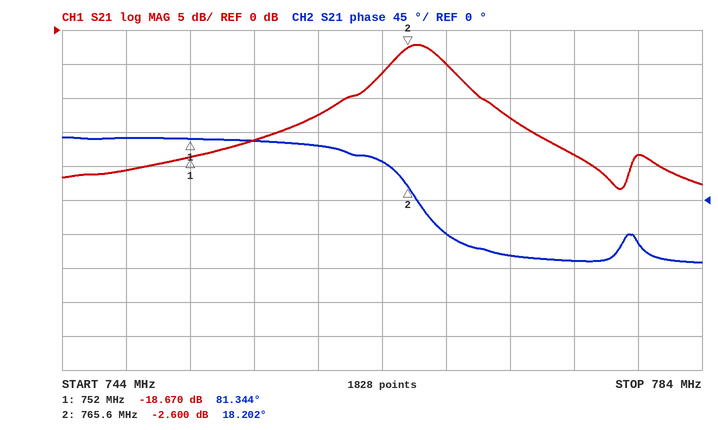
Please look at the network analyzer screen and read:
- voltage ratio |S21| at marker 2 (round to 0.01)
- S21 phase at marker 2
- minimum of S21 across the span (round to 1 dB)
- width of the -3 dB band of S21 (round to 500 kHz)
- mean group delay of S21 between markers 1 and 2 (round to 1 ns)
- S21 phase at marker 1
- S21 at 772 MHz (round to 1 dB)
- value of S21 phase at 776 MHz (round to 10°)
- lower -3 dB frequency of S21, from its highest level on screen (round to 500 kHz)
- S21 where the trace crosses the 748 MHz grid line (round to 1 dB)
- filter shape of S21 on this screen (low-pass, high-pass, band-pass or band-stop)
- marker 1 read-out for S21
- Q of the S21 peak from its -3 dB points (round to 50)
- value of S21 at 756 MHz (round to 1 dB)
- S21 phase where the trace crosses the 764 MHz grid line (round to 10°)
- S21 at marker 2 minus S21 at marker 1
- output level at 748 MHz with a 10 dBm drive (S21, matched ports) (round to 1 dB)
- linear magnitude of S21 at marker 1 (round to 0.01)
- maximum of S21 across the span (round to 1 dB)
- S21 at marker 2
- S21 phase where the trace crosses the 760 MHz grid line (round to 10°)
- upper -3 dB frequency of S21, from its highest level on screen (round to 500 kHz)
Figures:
0.74
18.202°
-23 dB
3.5 MHz
13 ns
81.344°
-13 dB
-80°
764.5 MHz
-21 dB
band-pass
-18.670 dB
200
-16 dB
50°
16.070 dB
-11 dBm
0.12
-2 dB
-2.600 dB
70°
768.0 MHz
